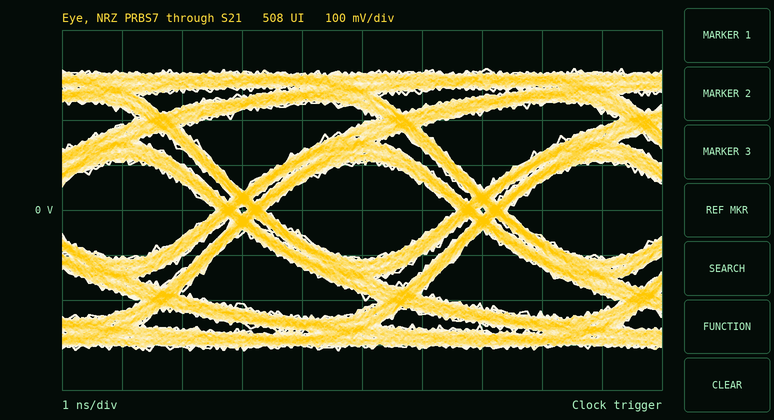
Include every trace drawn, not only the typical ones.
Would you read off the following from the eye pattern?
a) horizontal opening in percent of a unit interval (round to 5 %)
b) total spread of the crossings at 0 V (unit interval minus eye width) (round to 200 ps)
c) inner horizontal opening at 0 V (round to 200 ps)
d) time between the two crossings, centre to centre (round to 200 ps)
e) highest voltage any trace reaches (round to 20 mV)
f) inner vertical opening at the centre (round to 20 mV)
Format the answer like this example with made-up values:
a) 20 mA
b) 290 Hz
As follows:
a) 80 %
b) 800 ps
c) 3.2 ns
d) 4.0 ns
e) 320 mV
f) 220 mV
